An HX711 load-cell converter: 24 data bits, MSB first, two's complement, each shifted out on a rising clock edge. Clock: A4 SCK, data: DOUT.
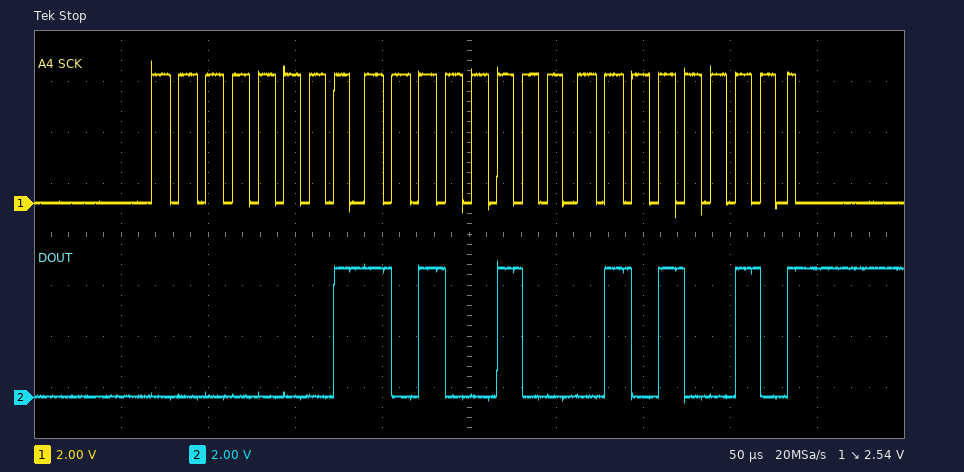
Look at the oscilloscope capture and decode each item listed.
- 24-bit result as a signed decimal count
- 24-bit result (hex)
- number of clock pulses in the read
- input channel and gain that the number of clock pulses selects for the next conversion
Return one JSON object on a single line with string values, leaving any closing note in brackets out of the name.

{"24-bit result as a signed decimal count": "107602", "24-bit result": "0x01A452", "number of clock pulses in the read": "25", "input channel and gain that the number of clock pulses selects for the next conversion": "channel A, gain 128"}
